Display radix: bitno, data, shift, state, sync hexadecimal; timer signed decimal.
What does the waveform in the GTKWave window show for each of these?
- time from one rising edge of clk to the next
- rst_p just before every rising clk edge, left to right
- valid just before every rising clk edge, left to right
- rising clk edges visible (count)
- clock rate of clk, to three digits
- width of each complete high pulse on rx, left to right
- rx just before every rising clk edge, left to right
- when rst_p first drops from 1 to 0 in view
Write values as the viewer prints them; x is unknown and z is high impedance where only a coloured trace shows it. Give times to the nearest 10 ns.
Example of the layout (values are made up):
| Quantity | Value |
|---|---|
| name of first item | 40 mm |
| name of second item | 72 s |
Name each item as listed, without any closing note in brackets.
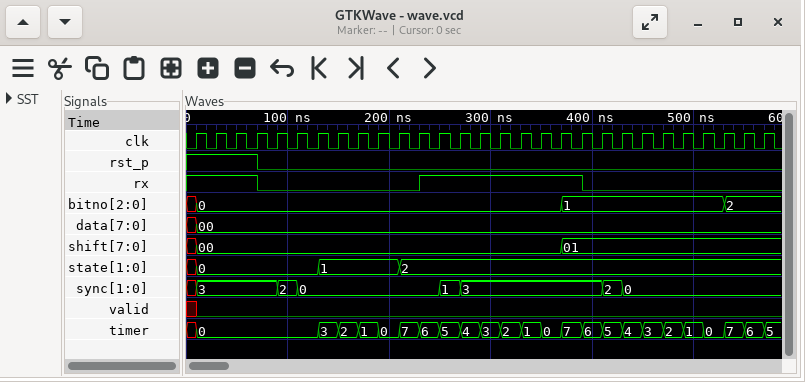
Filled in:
| Quantity | Value |
|---|---|
| time from one rising edge of clk to the next | 20 ns |
| rst_p just before every rising clk edge, left to right | 1 1 1 1 0 0 0 0 0 0 0 0 0 0 0 0 0 0 0 0 0 0 0 0 0 0 0 0 0 |
| valid just before every rising clk edge, left to right | x 0 0 0 0 0 0 0 0 0 0 0 0 0 0 0 0 0 0 0 0 0 0 0 0 0 0 0 0 |
| rising clk edges visible | 29 |
| clock rate of clk, to three digits | 50.0 MHz |
| width of each complete high pulse on rx, left to right | 160 ns |
| rx just before every rising clk edge, left to right | 1 1 1 1 0 0 0 0 0 0 0 0 1 1 1 1 1 1 1 1 0 0 0 0 0 0 0 0 0 |
| when rst_p first drops from 1 to 0 in view | 70 ns |
